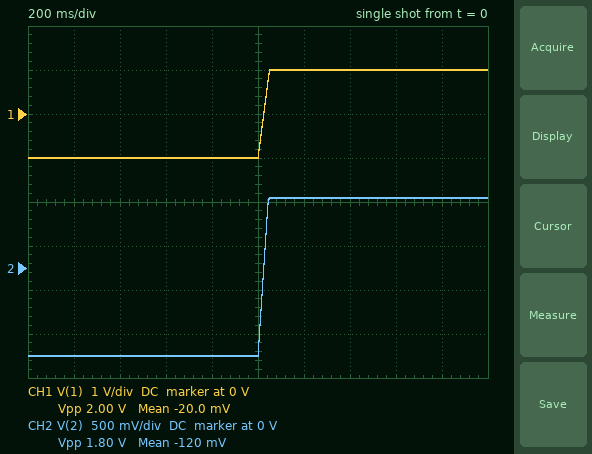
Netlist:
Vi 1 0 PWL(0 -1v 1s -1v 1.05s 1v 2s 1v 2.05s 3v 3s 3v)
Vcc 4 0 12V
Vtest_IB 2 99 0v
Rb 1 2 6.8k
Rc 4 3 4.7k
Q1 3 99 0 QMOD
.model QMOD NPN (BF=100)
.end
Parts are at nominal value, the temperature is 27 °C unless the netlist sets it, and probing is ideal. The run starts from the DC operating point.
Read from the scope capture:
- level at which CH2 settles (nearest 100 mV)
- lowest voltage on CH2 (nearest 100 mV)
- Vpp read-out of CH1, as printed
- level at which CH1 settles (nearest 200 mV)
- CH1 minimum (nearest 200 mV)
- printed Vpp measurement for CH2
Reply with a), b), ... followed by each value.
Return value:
a) 800 mV
b) -1.0 V
c) 2.00 V
d) 1.0 V
e) -1.0 V
f) 1.80 V
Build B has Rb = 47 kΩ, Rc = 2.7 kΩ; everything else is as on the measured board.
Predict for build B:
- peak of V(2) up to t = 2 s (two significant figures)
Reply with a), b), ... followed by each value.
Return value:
a) 760 mV
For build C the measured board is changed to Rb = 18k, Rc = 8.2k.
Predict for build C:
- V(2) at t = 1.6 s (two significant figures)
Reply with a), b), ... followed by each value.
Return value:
a) 780 mV
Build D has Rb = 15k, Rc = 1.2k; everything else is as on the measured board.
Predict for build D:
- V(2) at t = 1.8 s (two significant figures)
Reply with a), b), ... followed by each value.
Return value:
a) 780 mV
